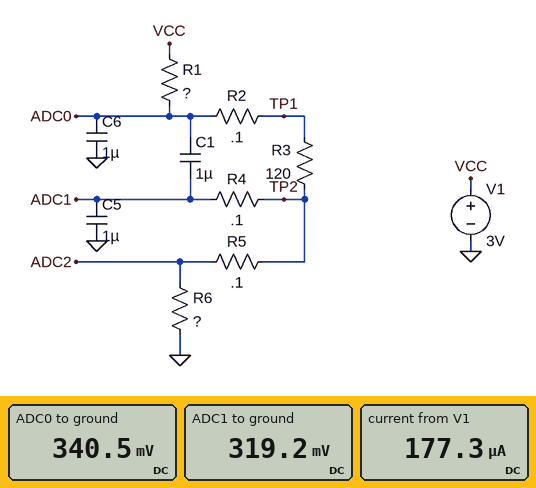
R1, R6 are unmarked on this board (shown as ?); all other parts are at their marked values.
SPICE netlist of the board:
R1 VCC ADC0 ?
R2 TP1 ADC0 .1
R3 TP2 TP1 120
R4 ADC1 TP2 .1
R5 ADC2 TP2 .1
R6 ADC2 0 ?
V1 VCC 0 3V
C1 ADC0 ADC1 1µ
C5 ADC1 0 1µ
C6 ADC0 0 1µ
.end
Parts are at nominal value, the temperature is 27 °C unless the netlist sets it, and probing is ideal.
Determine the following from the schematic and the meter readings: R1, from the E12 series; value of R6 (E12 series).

15 kΩ
1.8 kΩ
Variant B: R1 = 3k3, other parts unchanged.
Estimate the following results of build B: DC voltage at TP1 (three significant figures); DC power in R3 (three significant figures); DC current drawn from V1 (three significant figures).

1.10 V
39.6 µW
575 µA
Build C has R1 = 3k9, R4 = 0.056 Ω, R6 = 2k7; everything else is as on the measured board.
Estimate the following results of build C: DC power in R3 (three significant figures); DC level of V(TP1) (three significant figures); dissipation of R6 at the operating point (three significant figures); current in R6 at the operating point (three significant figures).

23.9 µW
1.26 V
538 µW
446 µA
